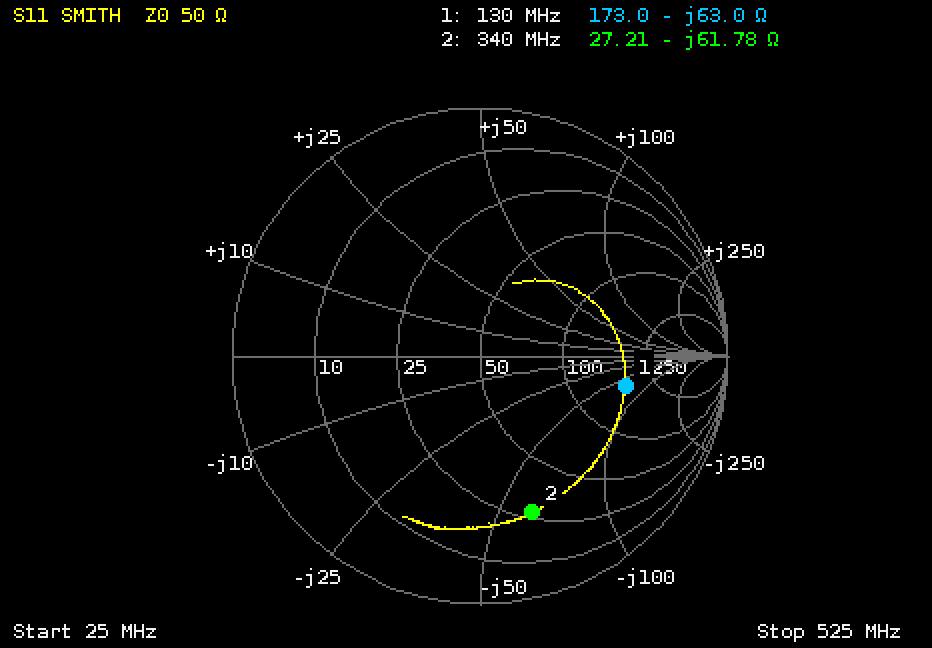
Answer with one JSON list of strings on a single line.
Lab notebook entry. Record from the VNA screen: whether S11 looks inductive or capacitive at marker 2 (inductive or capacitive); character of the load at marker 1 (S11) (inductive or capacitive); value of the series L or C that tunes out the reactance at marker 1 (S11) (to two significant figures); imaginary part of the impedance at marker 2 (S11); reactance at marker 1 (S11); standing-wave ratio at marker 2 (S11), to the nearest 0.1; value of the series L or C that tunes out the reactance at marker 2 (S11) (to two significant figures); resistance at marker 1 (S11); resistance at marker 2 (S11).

["capacitive", "capacitive", "77 nH", "-61.78 Ω", "-63.0 Ω", "5.0", "29 nH", "173.0 Ω", "27.21 Ω"]
